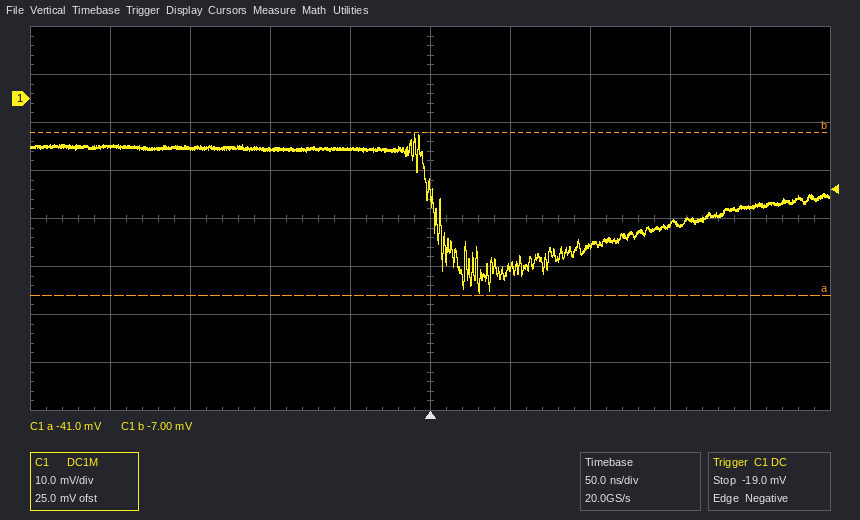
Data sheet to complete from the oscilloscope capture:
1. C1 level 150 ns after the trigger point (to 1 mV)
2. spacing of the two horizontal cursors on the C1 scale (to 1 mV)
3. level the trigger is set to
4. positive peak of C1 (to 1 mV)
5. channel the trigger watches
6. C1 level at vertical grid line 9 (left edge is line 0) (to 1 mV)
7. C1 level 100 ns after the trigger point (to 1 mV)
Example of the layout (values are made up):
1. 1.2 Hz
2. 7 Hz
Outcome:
1. -26 mV
2. 34 mV
3. -19.0 mV
4. -7 mV
5. C1
6. -23 mV
7. -31 mV
